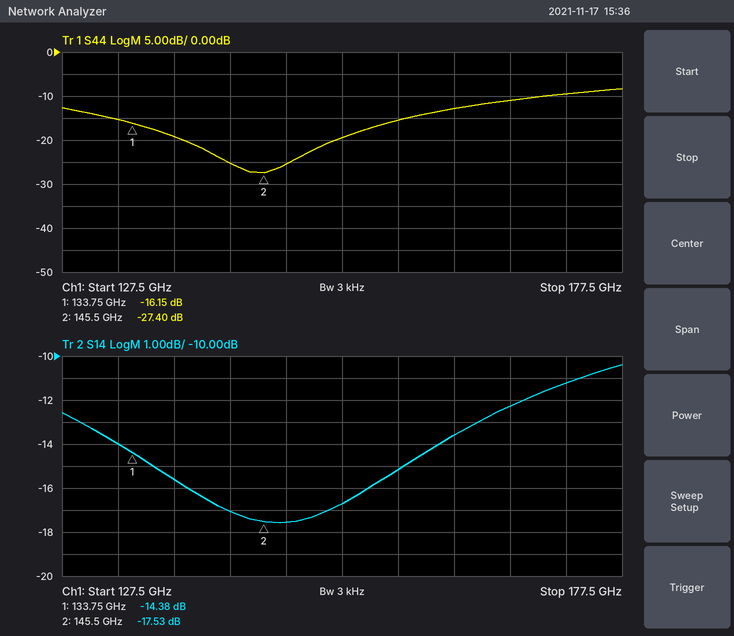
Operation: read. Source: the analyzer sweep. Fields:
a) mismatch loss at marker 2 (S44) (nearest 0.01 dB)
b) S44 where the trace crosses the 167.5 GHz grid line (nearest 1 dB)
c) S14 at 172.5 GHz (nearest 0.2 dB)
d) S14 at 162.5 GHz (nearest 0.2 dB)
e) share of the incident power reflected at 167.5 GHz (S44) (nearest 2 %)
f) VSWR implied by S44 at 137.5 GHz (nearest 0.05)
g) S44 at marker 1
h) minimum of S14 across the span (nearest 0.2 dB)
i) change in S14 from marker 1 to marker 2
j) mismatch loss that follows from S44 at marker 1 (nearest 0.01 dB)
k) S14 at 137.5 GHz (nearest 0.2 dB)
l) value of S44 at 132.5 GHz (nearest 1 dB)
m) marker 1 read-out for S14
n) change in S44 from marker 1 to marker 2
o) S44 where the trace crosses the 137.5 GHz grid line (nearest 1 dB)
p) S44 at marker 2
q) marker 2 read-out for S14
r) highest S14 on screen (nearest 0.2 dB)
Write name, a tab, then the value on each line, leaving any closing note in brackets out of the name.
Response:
mismatch loss at marker 2 (S44)	0.01 dB
S44 where the trace crosses the 167.5 GHz grid line	-11 dB
S14 at 172.5 GHz	-11.2 dB
S14 at 162.5 GHz	-13.6 dB
share of the incident power reflected at 167.5 GHz (S44)	8 %
VSWR implied by S44 at 137.5 GHz	1.25
S44 at marker 1	-16.15 dB
minimum of S14 across the span	-17.6 dB
change in S14 from marker 1 to marker 2	-3.15 dB
mismatch loss that follows from S44 at marker 1	0.11 dB
S14 at 137.5 GHz	-15.6 dB
value of S44 at 132.5 GHz	-15 dB
marker 1 read-out for S14	-14.38 dB
change in S44 from marker 1 to marker 2	-11.25 dB
S44 where the trace crosses the 137.5 GHz grid line	-19 dB
S44 at marker 2	-27.40 dB
marker 2 read-out for S14	-17.53 dB
highest S14 on screen	-10.4 dB
